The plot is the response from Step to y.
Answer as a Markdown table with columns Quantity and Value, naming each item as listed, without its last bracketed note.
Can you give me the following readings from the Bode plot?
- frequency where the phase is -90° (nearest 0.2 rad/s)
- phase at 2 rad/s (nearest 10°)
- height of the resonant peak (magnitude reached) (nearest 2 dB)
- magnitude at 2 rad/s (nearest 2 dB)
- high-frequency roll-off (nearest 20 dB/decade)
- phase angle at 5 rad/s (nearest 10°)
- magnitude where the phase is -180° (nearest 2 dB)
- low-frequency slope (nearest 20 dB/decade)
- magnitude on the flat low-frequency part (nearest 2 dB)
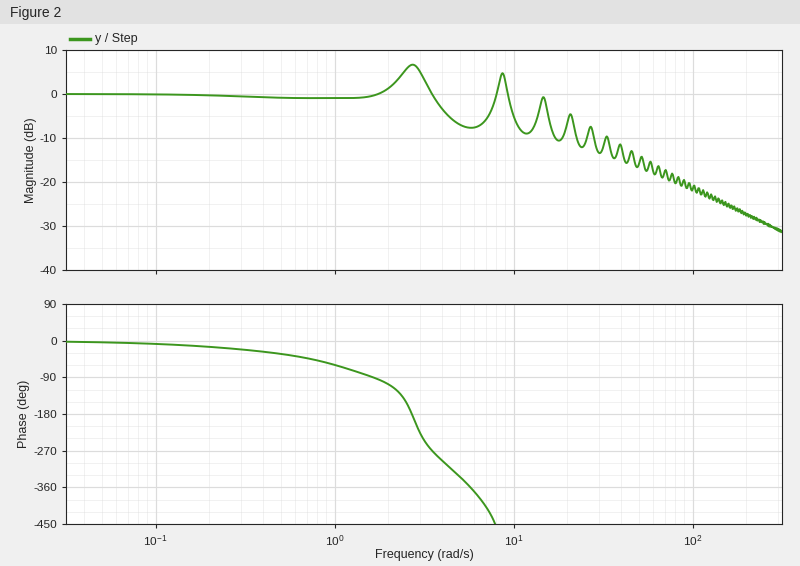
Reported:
| Quantity | Value |
|---|---|
| frequency where the phase is -90° | 1.6 rad/s |
| phase at 2 rad/s | -110° |
| height of the resonant peak (magnitude reached) | 6 dB |
| magnitude at 2 rad/s | 2 dB |
| high-frequency roll-off | -20 dB/decade |
| phase angle at 5 rad/s | -330° |
| magnitude where the phase is -180° | 6 dB |
| low-frequency slope | 0 dB/decade |
| magnitude on the flat low-frequency part | 0 dB |
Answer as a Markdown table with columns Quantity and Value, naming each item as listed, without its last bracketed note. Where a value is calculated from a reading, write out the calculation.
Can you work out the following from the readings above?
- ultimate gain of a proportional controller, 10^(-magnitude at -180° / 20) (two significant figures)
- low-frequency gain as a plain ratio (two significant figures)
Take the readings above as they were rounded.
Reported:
| Quantity | Value |
|---|---|
| ultimate gain of a proportional controller, 10^(-magnitude at -180° / 20) | 10^(-6 / 20) = 0.50 |
| low-frequency gain as a plain ratio | 10^(0 / 20) = 1.0 |
